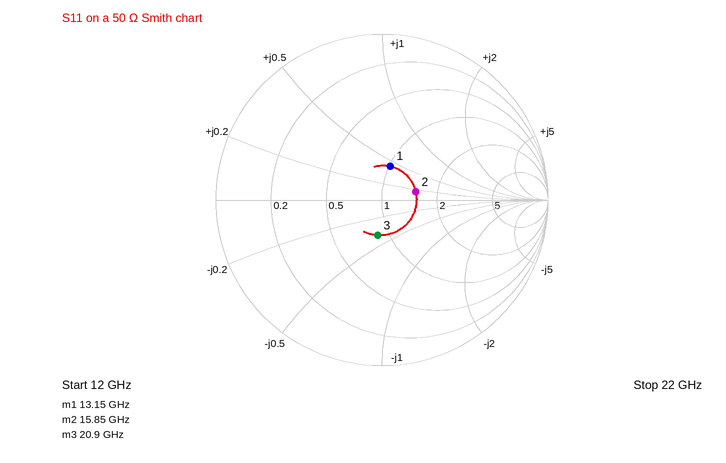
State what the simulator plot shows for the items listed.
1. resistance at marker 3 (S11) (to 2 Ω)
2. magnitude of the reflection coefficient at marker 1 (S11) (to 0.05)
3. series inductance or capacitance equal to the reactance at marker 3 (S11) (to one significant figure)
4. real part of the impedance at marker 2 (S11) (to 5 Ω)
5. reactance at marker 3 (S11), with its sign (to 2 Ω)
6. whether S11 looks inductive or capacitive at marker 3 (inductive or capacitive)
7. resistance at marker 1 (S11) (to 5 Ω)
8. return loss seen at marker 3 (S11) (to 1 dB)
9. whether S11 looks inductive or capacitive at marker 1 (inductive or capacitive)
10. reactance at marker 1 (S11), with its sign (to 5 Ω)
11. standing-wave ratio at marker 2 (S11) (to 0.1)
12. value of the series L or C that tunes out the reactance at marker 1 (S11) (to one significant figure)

44 Ω
0.20
400 fF
75 Ω
-20 Ω
capacitive
50 Ω
13 dB
inductive
+20 Ω
1.5
600 fF
